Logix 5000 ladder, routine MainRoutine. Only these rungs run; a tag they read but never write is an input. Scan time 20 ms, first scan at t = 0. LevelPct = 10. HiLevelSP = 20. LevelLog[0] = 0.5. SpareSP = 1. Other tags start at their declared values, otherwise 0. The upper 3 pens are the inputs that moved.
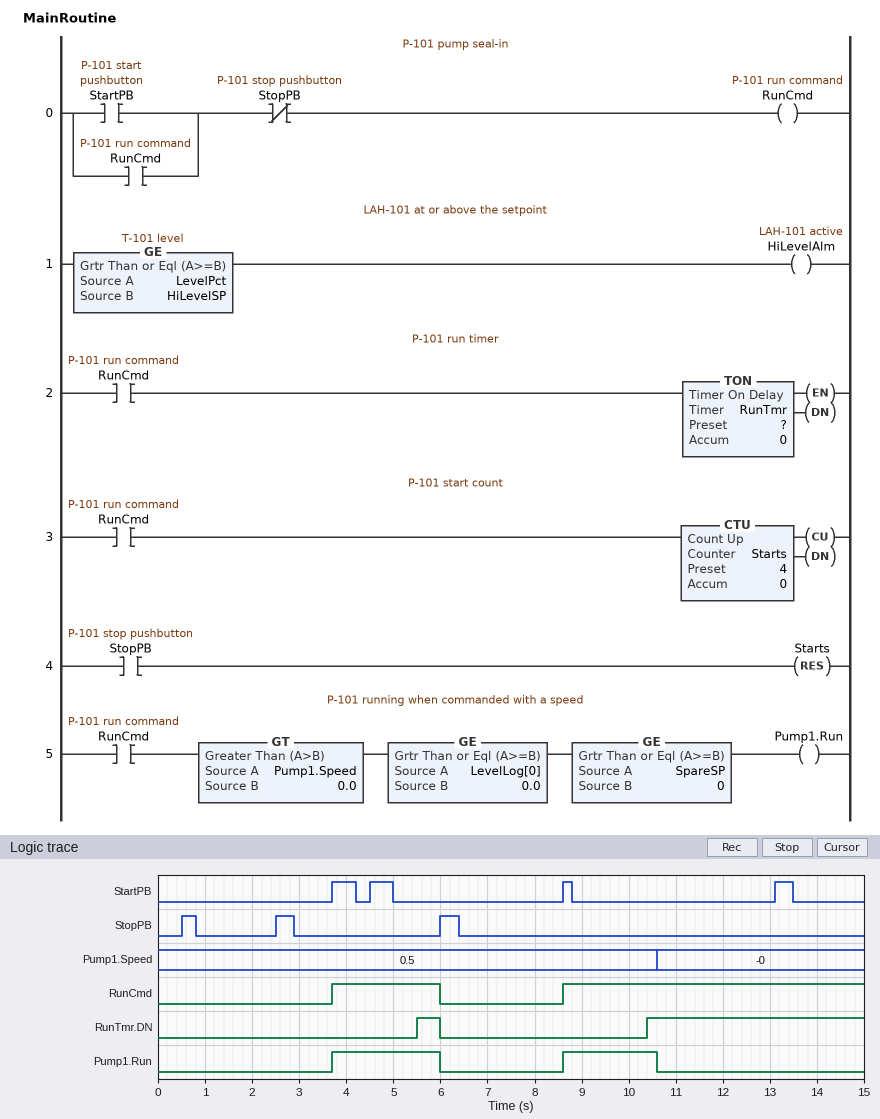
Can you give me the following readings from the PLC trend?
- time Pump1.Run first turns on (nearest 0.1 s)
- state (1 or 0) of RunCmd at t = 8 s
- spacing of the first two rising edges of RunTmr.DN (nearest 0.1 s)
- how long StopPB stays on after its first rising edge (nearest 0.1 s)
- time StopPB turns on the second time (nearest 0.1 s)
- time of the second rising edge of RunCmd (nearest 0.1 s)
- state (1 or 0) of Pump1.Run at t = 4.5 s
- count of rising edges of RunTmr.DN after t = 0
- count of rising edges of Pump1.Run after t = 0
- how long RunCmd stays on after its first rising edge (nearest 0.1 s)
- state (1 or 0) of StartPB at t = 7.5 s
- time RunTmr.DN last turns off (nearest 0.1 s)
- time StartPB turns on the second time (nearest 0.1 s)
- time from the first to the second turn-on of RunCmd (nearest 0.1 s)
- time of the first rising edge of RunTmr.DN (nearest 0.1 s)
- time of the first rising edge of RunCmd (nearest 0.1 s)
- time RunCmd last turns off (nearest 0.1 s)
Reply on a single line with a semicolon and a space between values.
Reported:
3.7 s; 0; 4.9 s; 0.3 s; 2.5 s; 8.6 s; 1; 2; 2; 2.3 s; 0; 6.0 s; 4.5 s; 4.9 s; 5.5 s; 3.7 s; 6.0 s
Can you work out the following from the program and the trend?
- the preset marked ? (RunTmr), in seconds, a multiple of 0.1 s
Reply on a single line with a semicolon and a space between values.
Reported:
1.8 s
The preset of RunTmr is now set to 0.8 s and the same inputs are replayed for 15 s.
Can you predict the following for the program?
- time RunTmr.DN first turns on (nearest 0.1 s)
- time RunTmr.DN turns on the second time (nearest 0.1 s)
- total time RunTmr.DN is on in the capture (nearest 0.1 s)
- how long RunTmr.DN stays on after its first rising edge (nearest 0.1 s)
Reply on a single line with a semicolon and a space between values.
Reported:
4.5 s; 9.4 s; 7.1 s; 1.5 s
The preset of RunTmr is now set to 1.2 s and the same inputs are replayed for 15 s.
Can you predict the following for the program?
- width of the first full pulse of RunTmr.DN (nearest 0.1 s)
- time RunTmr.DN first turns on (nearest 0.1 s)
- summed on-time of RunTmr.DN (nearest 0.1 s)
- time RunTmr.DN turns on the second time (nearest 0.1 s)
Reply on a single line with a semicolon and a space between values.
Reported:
1.1 s; 4.9 s; 6.3 s; 9.8 s
